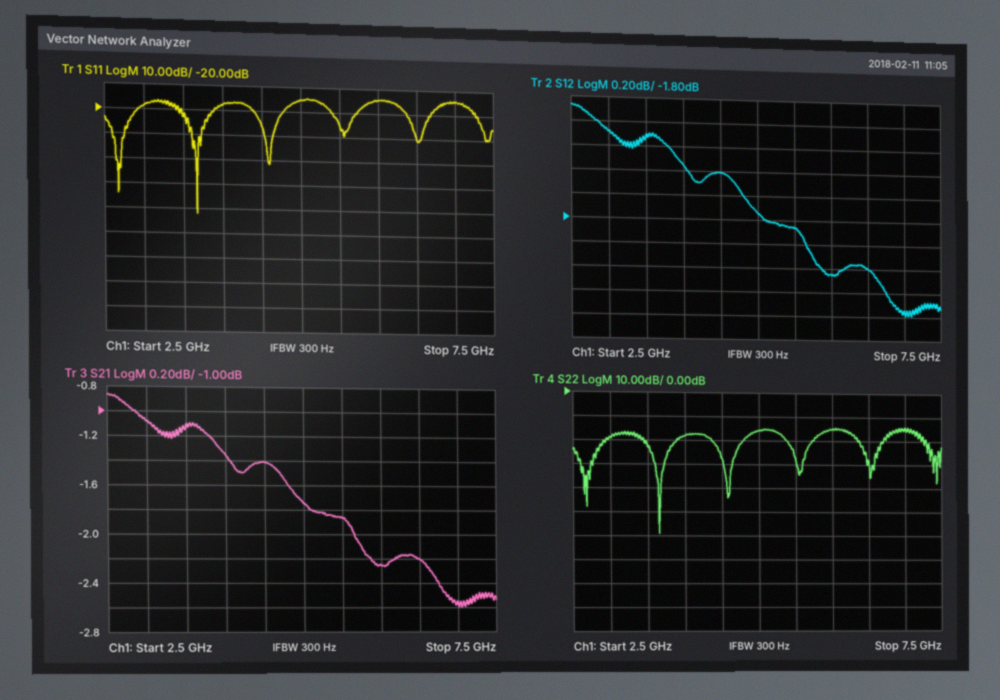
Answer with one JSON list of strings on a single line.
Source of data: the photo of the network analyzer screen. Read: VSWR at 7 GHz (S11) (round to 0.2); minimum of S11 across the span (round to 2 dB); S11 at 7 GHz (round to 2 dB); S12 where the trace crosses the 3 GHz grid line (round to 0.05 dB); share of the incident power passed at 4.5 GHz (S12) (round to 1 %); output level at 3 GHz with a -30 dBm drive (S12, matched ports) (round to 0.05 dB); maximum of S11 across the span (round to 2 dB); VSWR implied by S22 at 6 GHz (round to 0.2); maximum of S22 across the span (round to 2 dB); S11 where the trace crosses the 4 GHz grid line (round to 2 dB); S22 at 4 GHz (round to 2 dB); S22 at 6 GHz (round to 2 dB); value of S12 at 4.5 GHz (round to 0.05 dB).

["1.4", "-62 dB", "-14 dB", "-1.10 dB", "72 %", "-31.10 dBm", "-14 dB", "1.4", "-14 dB", "-18 dB", "-18 dB", "-16 dB", "-1.40 dB"]
